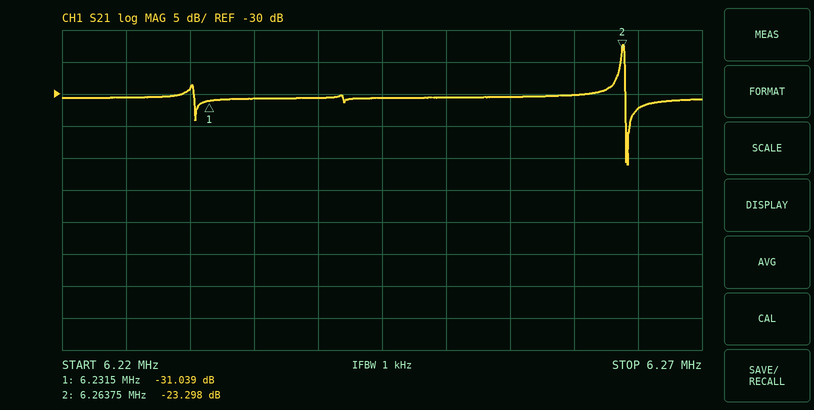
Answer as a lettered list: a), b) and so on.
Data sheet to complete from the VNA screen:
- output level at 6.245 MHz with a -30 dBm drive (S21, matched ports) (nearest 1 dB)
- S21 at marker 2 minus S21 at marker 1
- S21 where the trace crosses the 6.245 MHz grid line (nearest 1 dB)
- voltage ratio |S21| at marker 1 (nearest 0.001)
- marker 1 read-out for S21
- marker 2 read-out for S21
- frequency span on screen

a) -61 dBm
b) 7.741 dB
c) -31 dB
d) 0.028
e) -31.039 dB
f) -23.298 dB
g) 50 kHz
